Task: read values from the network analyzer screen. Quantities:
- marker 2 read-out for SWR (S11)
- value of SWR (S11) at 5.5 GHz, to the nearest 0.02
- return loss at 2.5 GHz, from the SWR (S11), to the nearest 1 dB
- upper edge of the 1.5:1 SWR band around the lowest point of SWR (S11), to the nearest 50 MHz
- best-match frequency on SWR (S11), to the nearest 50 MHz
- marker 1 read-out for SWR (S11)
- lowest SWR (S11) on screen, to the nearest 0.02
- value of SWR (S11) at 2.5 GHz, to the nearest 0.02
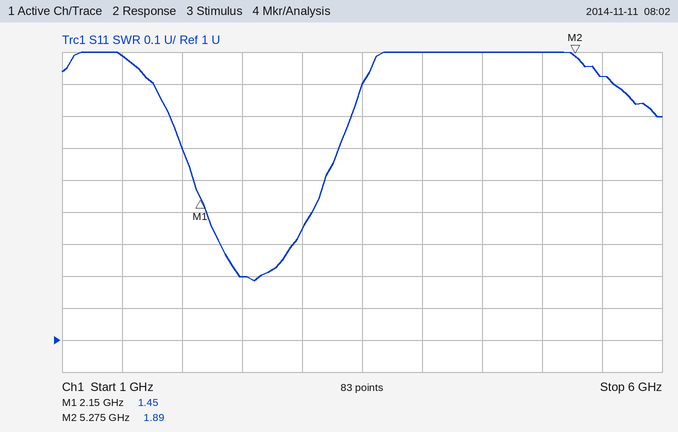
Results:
1.89
1.82
21 dB
3.20 GHz
2.60 GHz
1.45
1.18
1.20
